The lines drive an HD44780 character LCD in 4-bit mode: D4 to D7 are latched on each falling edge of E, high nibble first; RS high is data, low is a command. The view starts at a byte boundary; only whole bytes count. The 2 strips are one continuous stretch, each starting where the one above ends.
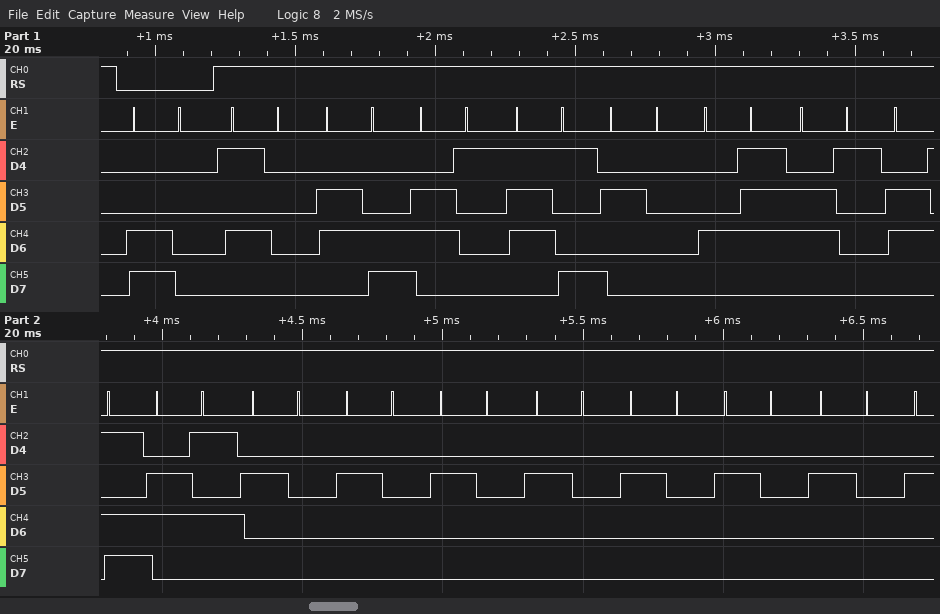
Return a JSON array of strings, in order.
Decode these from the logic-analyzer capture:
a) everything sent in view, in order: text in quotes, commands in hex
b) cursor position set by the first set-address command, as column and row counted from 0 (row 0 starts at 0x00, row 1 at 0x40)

["0xC0 \"Play Game       \"", "column 0, row 1"]
